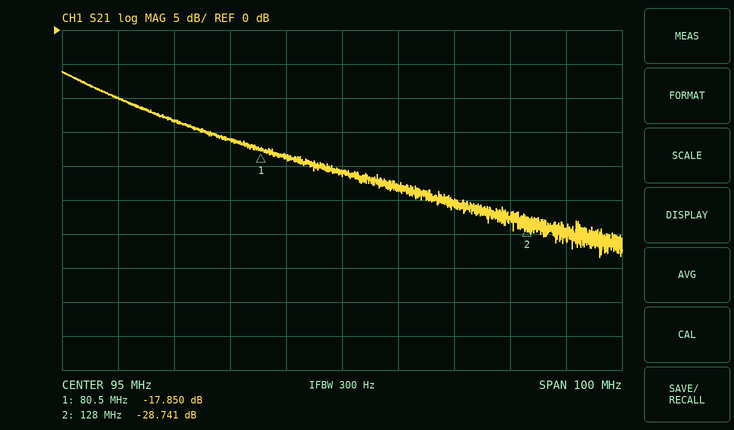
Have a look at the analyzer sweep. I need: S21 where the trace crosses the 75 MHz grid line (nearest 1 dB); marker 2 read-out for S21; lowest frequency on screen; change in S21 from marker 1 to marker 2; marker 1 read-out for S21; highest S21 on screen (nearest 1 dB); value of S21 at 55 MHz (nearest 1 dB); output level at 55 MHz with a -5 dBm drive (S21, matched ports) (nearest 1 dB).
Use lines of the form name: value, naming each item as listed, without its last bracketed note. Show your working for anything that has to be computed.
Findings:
S21 where the trace crosses the 75 MHz grid line: -16 dB
marker 2 read-out for S21: -28.741 dB
lowest frequency on screen: 45 MHz
change in S21 from marker 1 to marker 2: -28.741 − (-17.85) = -10.891 dB
marker 1 read-out for S21: -17.850 dB
highest S21 on screen: -6 dB
value of S21 at 55 MHz: -10 dB
output level at 55 MHz with a -5 dBm drive (S21, matched ports): -5 dBm + (-10 dB) = -15 dBm
